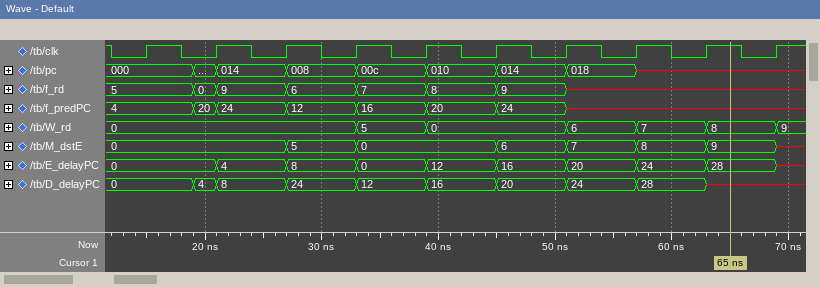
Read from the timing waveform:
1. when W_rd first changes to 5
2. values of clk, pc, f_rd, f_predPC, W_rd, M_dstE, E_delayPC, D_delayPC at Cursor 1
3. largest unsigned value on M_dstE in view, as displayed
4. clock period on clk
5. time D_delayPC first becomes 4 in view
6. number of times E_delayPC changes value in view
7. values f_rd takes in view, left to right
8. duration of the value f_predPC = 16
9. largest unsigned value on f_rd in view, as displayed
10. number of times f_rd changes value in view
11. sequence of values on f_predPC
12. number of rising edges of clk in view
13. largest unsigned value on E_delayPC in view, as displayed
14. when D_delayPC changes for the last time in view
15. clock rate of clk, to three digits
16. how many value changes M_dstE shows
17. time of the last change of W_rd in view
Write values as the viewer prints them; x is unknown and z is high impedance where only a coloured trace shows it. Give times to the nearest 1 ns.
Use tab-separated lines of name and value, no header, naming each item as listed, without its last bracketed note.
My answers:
when W_rd first changes to 5	33 ns
values of clk, pc, f_rd, f_predPC, W_rd, M_dstE, E_delayPC, D_delayPC at Cursor 1	clk=1, pc=x, f_rd=x, f_predPC=x, W_rd=8, M_dstE=9, E_delayPC=28, D_delayPC=x
largest unsigned value on M_dstE in view, as displayed	9
clock period on clk	6 ns
time D_delayPC first becomes 4 in view	19 ns
number of times E_delayPC changes value in view	9
values f_rd takes in view, left to right	5, 0, 9, 6, 7, 8, 9, x
duration of the value f_predPC = 16	6 ns
largest unsigned value on f_rd in view, as displayed	9
number of times f_rd changes value in view	7
sequence of values on f_predPC	4, 20, 24, 12, 16, 20, 24, x
number of rising edges of clk in view	10
largest unsigned value on E_delayPC in view, as displayed	28
when D_delayPC changes for the last time in view	63 ns
clock rate of clk, to three digits	167 MHz
how many value changes M_dstE shows	7
time of the last change of W_rd in view	69 ns
